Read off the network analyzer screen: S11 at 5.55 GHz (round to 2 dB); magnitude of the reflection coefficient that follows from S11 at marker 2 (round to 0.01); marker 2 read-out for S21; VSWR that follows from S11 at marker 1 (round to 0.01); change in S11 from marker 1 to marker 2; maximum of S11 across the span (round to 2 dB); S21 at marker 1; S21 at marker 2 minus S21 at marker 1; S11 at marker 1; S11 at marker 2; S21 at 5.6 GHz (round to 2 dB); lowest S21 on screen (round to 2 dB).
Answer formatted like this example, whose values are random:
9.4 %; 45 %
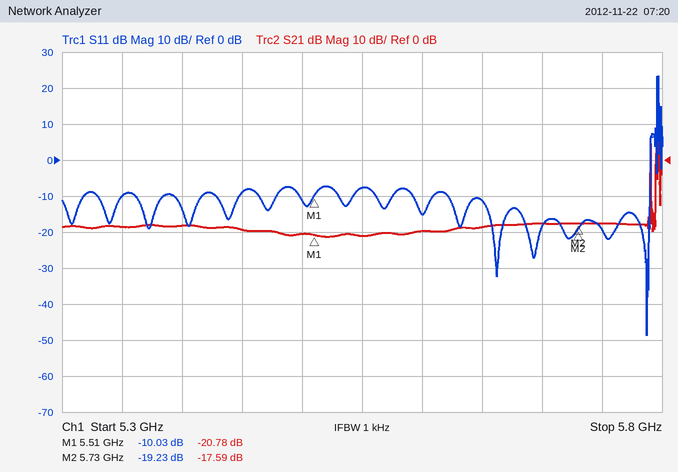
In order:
-8 dB; 0.11; -17.59 dB; 1.92; -9.20 dB; 24 dB; -20.78 dB; 3.19 dB; -10.03 dB; -19.23 dB; -20 dB; -22 dB
